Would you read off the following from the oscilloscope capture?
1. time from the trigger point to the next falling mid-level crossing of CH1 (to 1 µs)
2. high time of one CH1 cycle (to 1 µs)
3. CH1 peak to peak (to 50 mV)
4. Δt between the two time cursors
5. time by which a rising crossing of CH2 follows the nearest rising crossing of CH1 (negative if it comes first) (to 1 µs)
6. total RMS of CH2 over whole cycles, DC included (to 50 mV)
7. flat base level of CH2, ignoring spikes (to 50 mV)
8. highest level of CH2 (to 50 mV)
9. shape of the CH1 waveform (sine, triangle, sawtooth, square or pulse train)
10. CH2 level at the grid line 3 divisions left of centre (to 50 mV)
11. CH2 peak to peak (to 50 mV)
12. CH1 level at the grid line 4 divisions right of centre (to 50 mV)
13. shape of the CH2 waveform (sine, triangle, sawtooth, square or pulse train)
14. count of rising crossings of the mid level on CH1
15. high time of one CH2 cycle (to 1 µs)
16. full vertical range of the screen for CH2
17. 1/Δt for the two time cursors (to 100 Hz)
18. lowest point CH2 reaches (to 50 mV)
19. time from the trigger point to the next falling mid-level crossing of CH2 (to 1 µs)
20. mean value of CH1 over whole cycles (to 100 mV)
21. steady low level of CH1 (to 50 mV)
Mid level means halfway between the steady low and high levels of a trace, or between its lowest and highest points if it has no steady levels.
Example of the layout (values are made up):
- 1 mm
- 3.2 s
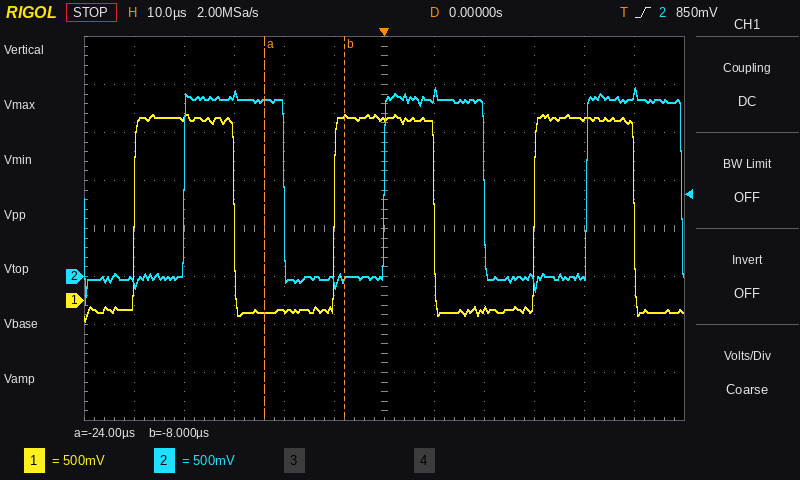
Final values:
- 10 µs
- 20 µs
- 2.15 V
- 16 µs
- +10 µs
- 1.30 V
- 0 mV
- 1.95 V
- square
- 1.90 V
- 2.25 V
- 1.90 V
- square
- 3
- 20 µs
- 4 V
- 62.5 kHz
- -300 mV
- 20 µs
- 900 mV
- -100 mV
